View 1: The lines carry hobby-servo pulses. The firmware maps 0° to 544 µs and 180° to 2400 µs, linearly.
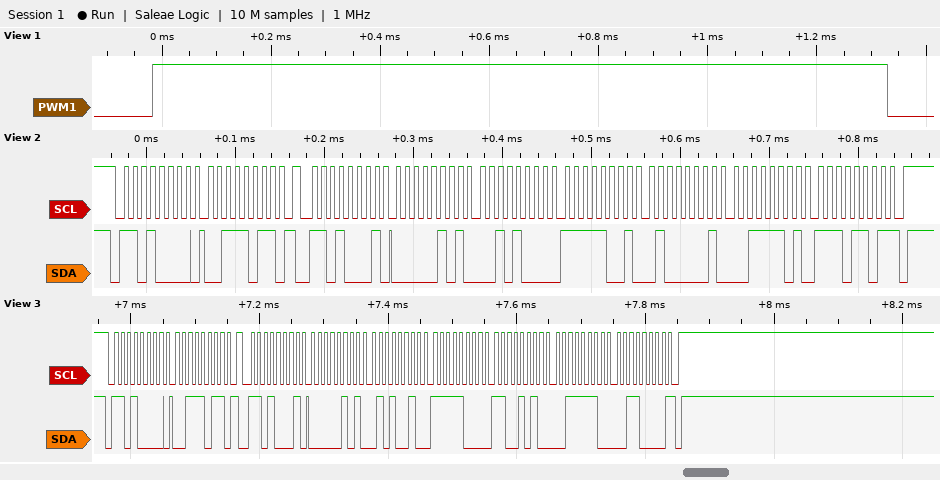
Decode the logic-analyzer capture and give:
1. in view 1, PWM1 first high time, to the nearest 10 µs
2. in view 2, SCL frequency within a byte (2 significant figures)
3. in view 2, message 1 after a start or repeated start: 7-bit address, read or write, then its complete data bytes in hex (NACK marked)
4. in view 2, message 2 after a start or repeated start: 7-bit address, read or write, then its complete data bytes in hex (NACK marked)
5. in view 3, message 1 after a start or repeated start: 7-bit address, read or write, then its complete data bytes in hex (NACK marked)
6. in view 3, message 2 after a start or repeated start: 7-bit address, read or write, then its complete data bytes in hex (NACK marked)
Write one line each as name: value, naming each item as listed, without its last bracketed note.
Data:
in view 1, PWM1 first high time, to the nearest 10 µs: 1350 µs
in view 2, SCL frequency within a byte: 100 kHz
in view 2, message 1 after a start or repeated start: 7-bit address, read or write, then its complete data bytes in hex: 0x68 write: 3B
in view 2, message 2 after a start or repeated start: 7-bit address, read or write, then its complete data bytes in hex: 0x68 read: 05 28 F9 41 3D ED NACK
in view 3, message 1 after a start or repeated start: 7-bit address, read or write, then its complete data bytes in hex: 0x68 write: 3B
in view 3, message 2 after a start or repeated start: 7-bit address, read or write, then its complete data bytes in hex: 0x68 read: 05 52 F8 CA 3E 30 NACK
